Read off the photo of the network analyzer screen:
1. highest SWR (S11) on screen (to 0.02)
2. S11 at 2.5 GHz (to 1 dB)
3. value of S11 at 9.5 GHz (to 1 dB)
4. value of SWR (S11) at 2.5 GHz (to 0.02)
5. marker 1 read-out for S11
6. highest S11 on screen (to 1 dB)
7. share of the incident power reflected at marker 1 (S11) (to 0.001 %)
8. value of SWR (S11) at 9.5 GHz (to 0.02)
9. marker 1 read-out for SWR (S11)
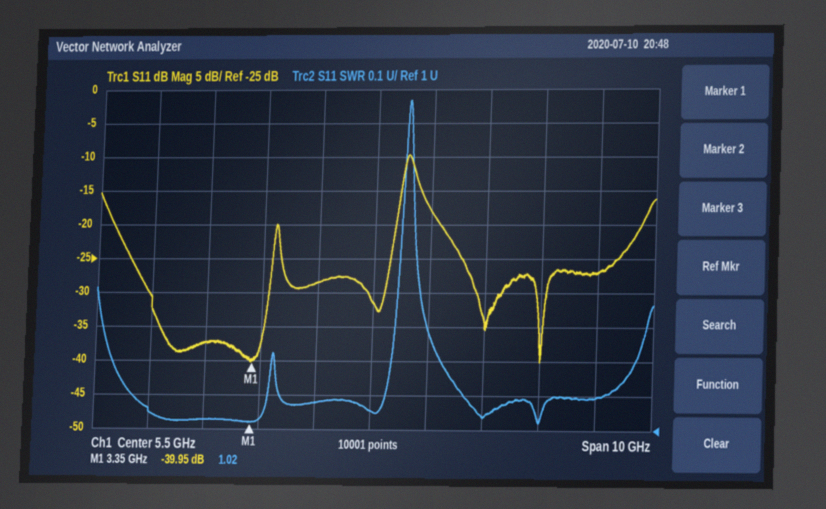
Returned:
1.96
-37 dB
-27 dB
1.02
-39.95 dB
-10 dB
0.010 %
1.10
1.02
